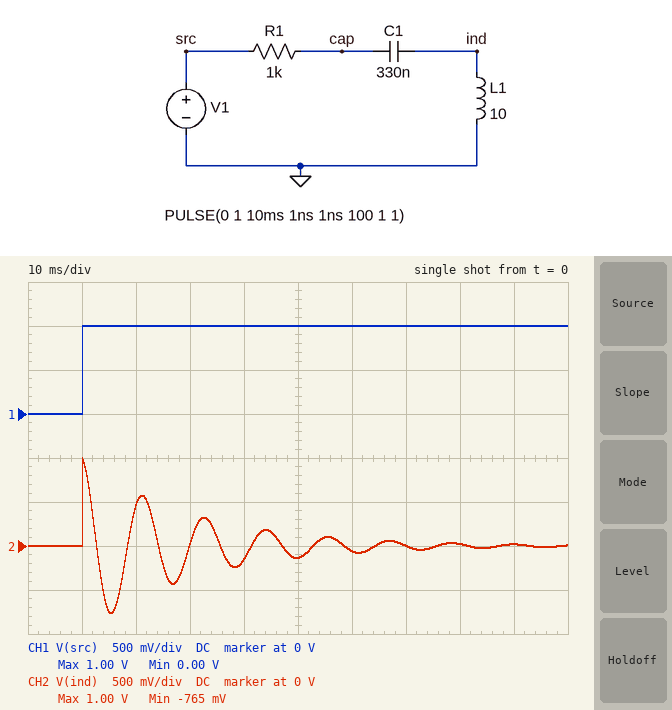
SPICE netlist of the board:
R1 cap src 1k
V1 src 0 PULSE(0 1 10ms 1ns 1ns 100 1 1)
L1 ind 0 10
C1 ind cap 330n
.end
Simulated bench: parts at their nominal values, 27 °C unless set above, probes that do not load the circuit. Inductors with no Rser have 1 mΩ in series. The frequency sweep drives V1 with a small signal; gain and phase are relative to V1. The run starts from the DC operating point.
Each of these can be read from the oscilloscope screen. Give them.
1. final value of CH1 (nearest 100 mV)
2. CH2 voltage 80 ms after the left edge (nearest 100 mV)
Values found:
1.0 V
0 V
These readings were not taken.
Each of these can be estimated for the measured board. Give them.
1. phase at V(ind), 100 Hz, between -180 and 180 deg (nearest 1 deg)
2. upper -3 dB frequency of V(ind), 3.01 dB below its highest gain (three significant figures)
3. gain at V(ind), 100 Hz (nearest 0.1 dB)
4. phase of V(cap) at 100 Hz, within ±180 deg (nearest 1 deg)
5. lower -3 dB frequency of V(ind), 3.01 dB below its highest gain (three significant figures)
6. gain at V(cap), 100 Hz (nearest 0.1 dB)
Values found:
34 deg
97.8 Hz
11.0 dB
34 deg
81.2 Hz
-1.7 dB
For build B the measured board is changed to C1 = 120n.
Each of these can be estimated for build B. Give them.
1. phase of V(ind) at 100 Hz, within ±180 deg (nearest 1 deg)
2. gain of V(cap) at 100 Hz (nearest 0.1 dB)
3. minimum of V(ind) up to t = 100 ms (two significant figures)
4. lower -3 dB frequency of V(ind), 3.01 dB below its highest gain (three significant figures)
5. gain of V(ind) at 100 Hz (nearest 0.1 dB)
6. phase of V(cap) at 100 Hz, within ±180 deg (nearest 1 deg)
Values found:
172 deg
-0.1 dB
-850 mV
138 Hz
-1.0 dB
-8 deg
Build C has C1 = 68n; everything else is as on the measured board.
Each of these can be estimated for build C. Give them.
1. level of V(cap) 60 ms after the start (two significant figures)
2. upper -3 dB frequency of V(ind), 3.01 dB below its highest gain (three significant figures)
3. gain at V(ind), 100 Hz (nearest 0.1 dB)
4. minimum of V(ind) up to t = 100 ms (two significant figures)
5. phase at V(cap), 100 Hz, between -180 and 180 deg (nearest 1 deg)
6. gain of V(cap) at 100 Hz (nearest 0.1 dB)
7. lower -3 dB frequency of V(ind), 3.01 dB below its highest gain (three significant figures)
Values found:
1.0 V
202 Hz
-8.7 dB
-880 mV
-3 deg
0 dB
186 Hz
